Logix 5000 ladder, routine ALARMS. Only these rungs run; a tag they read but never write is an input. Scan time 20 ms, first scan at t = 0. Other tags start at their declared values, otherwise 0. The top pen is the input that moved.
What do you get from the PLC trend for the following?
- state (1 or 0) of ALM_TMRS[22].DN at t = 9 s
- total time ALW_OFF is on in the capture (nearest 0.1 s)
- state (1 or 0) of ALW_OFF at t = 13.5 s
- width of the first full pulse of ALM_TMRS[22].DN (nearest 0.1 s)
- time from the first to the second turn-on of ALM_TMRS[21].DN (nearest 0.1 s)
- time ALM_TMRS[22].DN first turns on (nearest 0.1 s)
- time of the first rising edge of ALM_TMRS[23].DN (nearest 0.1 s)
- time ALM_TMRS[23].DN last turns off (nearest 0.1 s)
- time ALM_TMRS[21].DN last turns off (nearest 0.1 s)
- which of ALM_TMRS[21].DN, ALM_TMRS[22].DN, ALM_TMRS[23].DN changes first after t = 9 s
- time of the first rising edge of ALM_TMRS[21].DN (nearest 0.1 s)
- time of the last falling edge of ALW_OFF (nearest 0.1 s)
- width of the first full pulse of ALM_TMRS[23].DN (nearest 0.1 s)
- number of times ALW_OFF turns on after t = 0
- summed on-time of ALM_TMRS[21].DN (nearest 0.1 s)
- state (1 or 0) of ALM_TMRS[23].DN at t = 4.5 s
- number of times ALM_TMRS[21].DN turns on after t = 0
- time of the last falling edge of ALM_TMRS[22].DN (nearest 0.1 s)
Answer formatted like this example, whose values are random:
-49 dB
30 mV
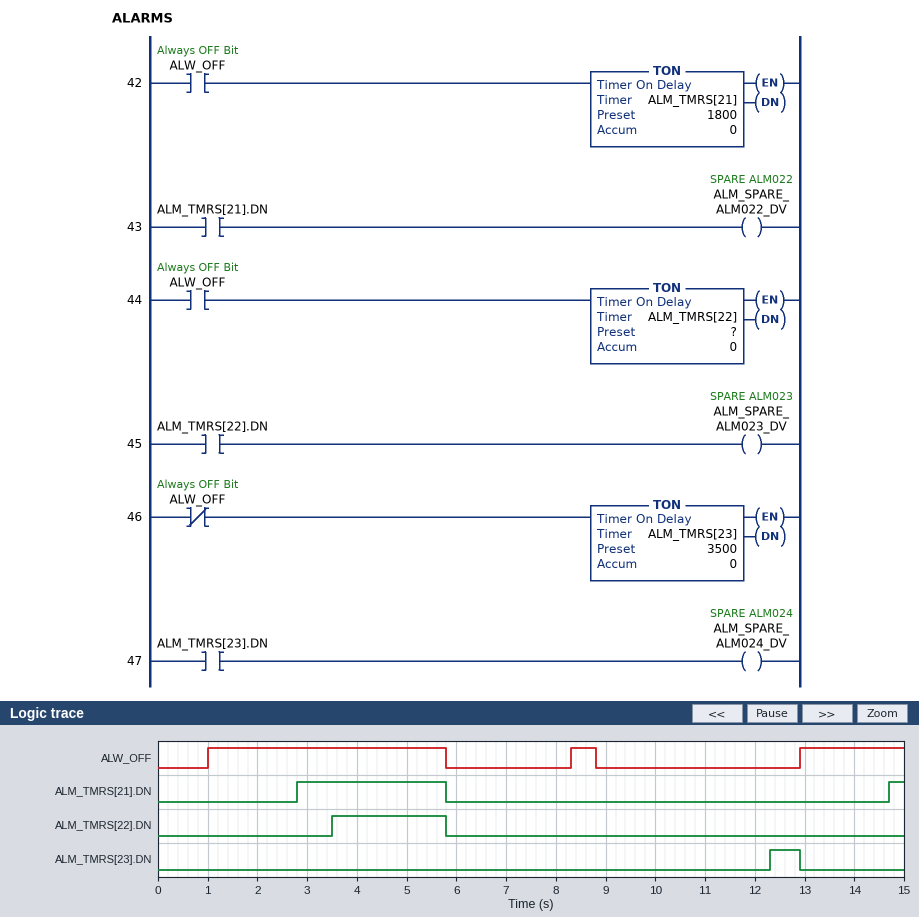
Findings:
0
7.4 s
1
2.3 s
11.9 s
3.5 s
12.3 s
12.9 s
5.8 s
ALM_TMRS[23].DN
2.8 s
8.8 s
0.6 s
3
3.3 s
0
2
5.8 s
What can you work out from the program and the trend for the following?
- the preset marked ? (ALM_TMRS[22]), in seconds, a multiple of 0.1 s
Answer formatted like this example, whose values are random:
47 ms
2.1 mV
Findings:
2.5 s
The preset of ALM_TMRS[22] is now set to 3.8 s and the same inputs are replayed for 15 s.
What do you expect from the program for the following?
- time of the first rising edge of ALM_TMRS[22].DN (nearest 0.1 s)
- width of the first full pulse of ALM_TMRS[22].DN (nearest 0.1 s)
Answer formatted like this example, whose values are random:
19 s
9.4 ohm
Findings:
4.8 s
1.0 s
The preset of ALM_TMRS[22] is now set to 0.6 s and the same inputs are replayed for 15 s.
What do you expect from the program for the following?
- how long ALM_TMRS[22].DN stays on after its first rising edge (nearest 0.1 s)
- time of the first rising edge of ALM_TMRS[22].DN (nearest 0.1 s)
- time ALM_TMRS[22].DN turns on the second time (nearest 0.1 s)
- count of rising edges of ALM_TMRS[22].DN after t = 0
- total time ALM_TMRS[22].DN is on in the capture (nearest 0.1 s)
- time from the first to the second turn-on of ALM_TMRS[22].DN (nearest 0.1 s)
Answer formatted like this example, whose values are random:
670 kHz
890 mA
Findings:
4.2 s
1.6 s
13.5 s
2
5.7 s
11.9 s
